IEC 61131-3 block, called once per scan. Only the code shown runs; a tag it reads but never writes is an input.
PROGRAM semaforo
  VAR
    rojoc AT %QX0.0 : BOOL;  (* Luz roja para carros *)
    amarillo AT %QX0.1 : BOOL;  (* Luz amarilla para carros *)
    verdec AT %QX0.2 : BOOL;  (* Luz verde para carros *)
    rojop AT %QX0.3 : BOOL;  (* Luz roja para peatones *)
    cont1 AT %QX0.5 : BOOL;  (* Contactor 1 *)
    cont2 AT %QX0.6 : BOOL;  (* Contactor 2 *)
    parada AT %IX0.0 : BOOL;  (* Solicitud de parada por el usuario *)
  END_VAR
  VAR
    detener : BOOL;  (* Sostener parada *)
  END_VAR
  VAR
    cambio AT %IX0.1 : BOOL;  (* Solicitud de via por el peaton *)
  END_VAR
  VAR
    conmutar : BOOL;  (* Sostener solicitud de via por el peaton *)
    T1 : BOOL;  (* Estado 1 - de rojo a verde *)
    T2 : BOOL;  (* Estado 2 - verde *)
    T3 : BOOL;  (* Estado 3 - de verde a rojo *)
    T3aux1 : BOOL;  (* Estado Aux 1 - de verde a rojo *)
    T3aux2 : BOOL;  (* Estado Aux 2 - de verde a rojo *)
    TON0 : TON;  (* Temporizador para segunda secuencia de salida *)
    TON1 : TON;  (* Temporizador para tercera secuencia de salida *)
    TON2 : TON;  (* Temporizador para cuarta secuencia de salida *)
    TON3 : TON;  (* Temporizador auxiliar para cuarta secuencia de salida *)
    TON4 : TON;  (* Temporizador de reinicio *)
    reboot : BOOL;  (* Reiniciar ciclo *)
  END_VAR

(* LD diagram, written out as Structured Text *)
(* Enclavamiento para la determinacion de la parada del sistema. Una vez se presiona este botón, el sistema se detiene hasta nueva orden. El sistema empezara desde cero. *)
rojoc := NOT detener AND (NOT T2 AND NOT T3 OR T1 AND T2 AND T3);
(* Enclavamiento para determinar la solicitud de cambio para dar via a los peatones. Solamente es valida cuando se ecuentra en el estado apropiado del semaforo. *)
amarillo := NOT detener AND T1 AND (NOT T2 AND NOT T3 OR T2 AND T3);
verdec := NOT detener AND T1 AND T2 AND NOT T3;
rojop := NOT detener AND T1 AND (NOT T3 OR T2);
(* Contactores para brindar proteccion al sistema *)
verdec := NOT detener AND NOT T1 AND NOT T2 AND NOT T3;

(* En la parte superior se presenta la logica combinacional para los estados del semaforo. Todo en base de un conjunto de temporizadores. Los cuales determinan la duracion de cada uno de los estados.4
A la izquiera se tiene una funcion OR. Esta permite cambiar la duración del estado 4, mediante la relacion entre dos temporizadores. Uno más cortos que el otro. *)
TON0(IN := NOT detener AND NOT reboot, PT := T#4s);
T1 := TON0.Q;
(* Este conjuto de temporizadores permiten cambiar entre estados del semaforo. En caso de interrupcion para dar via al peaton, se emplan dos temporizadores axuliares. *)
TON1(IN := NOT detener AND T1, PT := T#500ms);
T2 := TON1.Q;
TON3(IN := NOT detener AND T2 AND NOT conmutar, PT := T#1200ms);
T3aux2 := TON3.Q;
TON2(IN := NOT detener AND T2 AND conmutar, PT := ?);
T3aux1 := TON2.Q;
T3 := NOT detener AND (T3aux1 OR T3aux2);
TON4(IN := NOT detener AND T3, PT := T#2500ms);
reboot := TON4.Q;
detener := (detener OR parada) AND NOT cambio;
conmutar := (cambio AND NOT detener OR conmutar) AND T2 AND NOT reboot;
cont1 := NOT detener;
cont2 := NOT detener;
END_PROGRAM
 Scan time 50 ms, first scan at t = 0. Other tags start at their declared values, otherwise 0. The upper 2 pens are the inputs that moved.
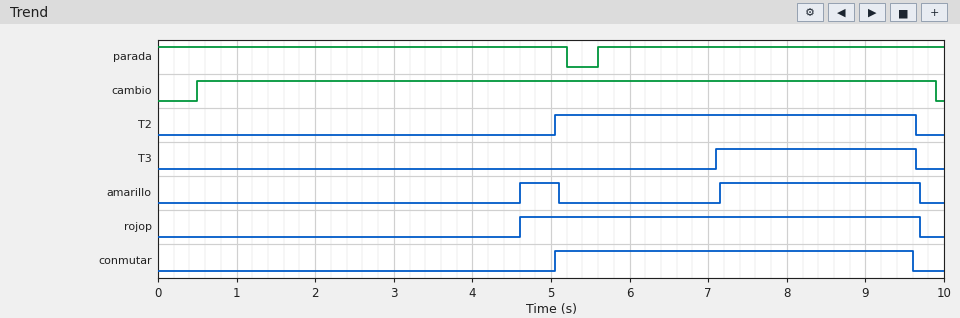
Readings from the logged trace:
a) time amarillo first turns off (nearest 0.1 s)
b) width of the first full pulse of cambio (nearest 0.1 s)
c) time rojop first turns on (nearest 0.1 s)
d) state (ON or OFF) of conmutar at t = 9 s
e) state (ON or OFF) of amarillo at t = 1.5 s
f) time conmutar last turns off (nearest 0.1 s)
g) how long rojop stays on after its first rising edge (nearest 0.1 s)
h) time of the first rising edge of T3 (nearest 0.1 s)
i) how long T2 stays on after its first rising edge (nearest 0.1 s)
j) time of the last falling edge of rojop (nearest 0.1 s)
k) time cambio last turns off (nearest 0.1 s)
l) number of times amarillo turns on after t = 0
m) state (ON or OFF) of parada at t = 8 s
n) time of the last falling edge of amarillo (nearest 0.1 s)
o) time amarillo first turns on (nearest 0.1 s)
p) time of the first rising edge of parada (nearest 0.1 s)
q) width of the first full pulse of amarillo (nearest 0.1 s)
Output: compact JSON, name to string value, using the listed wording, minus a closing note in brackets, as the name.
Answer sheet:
{"time amarillo first turns off": "5.1 s", "width of the first full pulse of cambio": "9.4 s", "time rojop first turns on": "4.6 s", "state (ON or OFF) of conmutar at t = 9 s": "ON", "state (ON or OFF) of amarillo at t = 1.5 s": "OFF", "time conmutar last turns off": "9.6 s", "how long rojop stays on after its first rising edge": "5.1 s", "time of the first rising edge of T3": "7.1 s", "how long T2 stays on after its first rising edge": "4.6 s", "time of the last falling edge of rojop": "9.7 s", "time cambio last turns off": "9.9 s", "number of times amarillo turns on after t = 0": "2", "state (ON or OFF) of parada at t = 8 s": "ON", "time of the last falling edge of amarillo": "9.7 s", "time amarillo first turns on": "4.6 s", "time of the first rising edge of parada": "5.6 s", "width of the first full pulse of amarillo": "0.5 s"}
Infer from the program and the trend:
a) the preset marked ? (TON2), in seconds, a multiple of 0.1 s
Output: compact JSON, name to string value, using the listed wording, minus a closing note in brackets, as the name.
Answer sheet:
{"the preset marked ? (TON2), in seconds, a multiple of 0.1 s": "2.0 s"}
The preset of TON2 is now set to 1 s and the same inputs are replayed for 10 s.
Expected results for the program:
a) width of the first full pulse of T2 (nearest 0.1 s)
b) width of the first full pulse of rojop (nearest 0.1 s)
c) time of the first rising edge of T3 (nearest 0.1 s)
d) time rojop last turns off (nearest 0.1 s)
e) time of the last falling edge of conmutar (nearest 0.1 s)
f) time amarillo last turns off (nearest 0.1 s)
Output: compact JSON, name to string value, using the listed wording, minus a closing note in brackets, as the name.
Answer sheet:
{"width of the first full pulse of T2": "3.6 s", "width of the first full pulse of rojop": "4.1 s", "time of the first rising edge of T3": "6.1 s", "time rojop last turns off": "8.7 s", "time of the last falling edge of conmutar": "8.6 s", "time amarillo last turns off": "8.7 s"}
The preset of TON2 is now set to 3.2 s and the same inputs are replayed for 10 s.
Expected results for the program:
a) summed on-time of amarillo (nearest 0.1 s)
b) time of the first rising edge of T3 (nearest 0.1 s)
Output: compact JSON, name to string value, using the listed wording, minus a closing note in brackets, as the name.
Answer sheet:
{"summed on-time of amarillo": "2.1 s", "time of the first rising edge of T3": "8.3 s"}
